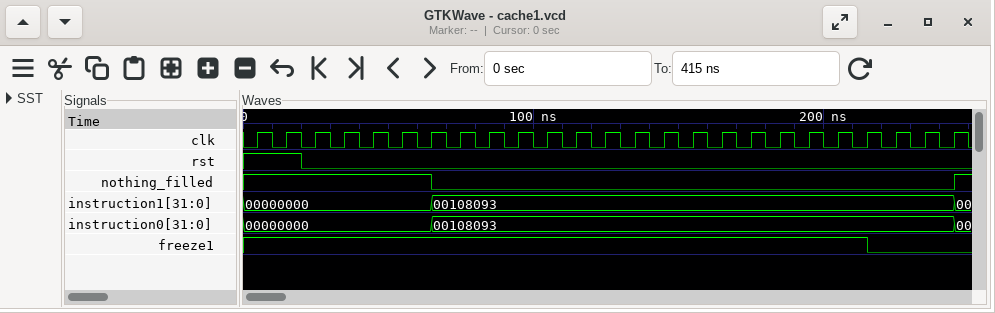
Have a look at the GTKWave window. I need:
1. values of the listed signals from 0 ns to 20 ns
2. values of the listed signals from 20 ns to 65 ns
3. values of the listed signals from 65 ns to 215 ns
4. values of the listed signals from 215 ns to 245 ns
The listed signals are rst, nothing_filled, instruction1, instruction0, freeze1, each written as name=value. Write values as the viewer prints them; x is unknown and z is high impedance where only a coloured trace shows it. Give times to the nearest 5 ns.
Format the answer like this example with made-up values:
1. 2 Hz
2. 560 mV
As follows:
1. rst=1, nothing_filled=1, instruction1=00000000, instruction0=00000000, freeze1=1
2. rst=0, nothing_filled=1, instruction1=00000000, instruction0=00000000, freeze1=1
3. rst=0, nothing_filled=0, instruction1=00108093, instruction0=00108093, freeze1=1
4. rst=0, nothing_filled=0, instruction1=00108093, instruction0=00108093, freeze1=0
